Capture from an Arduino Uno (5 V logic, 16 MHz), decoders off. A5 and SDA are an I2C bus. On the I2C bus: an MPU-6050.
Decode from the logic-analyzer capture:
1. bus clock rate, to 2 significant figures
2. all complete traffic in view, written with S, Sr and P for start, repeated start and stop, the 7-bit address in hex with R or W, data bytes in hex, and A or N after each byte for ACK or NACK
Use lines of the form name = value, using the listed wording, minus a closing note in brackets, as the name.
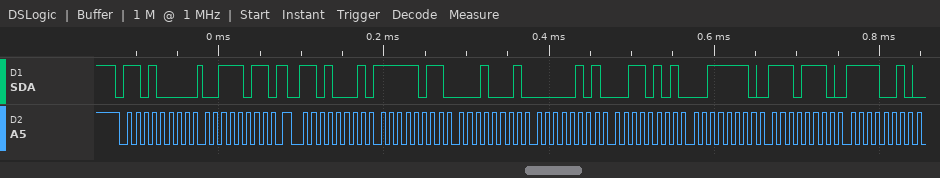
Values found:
bus clock rate, to 2 significant figures = 100 kHz
all complete traffic in view, written with S, Sr and P for start, repeated start and stop, the 7-bit address in hex with R or W, data bytes in hex, and A or N after each byte for ACK or NACK = S 68W A 3B A Sr 68R A FB A 11 A 05 A 35 A 3E A EE A F2 A
